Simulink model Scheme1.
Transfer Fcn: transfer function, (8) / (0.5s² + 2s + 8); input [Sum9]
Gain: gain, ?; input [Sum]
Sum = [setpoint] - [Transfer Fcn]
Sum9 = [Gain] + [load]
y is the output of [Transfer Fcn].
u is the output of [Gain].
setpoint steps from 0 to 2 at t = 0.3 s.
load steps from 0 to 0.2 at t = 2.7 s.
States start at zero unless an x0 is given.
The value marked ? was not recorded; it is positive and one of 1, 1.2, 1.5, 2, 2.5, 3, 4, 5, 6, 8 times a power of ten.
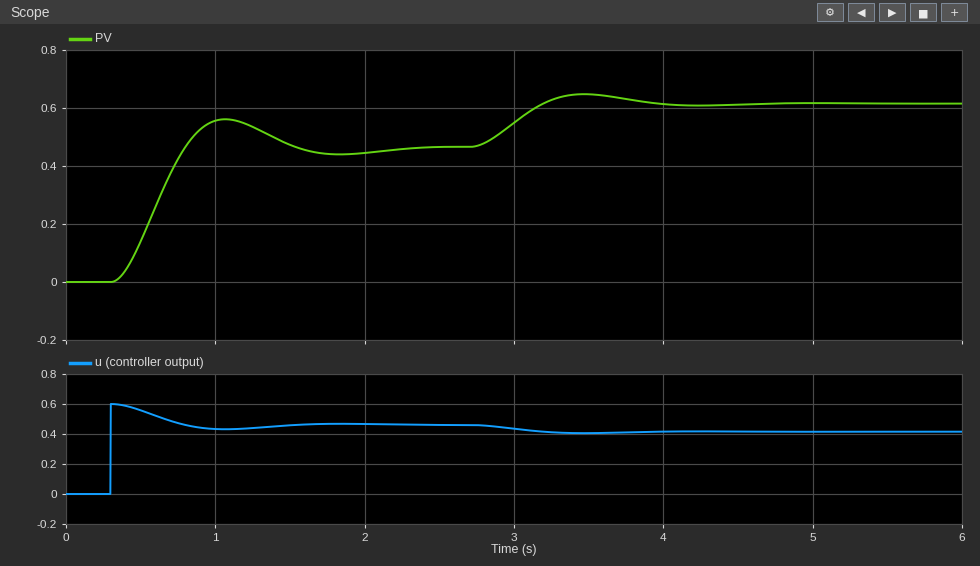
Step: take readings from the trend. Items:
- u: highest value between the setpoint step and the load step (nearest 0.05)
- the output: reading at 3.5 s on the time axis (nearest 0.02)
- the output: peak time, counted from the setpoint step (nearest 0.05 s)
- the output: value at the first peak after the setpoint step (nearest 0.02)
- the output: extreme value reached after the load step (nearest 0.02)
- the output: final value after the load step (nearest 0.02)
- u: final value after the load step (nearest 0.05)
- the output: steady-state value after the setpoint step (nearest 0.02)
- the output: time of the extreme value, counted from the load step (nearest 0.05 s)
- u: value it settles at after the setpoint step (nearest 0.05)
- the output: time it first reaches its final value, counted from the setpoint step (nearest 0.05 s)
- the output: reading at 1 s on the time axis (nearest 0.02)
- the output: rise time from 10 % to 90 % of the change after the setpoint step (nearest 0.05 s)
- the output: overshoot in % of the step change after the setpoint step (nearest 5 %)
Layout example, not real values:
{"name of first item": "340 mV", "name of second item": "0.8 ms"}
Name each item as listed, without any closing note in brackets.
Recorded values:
{"u: highest value between the setpoint step and the load step": "0.60", "the output: reading at 3.5 s on the time axis": "0.64", "the output: peak time, counted from the setpoint step": "0.75 s", "the output: value at the first peak after the setpoint step": "0.56", "the output: extreme value reached after the load step": "0.64", "the output: final value after the load step": "0.62", "u: final value after the load step": "0.40", "the output: steady-state value after the setpoint step": "0.46", "the output: time of the extreme value, counted from the load step": "0.75 s", "u: value it settles at after the setpoint step": "0.45", "the output: time it first reaches its final value, counted from the setpoint step": "0.50 s", "the output: reading at 1 s on the time axis": "0.56", "the output: rise time from 10 % to 90 % of the change after the setpoint step": "0.35 s", "the output: overshoot in % of the step change after the setpoint step": "20 %"}
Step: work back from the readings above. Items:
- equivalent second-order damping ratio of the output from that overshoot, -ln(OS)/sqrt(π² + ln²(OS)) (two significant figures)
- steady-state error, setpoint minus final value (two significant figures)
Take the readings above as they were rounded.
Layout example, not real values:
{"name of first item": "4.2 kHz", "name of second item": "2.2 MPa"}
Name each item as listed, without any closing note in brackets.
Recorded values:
{"equivalent second-order damping ratio of the output from that overshoot, -ln(OS)/sqrt(π² + ln²(OS))": "0.46", "steady-state error, setpoint minus final value": "1.5"}
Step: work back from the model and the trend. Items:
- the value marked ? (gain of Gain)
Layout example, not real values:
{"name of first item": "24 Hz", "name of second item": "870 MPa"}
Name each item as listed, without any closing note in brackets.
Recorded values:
{"the value marked ?": "0.3"}
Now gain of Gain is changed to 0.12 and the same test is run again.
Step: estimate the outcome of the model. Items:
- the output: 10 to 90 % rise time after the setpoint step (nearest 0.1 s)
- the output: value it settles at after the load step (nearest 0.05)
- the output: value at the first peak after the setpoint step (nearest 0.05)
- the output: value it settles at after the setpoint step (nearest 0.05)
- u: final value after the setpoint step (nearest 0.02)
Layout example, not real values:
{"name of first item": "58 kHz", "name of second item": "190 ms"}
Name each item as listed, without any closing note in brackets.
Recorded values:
{"the output: 10 to 90 % rise time after the setpoint step": "0.4 s", "the output: value it settles at after the load step": "0.40", "the output: value at the first peak after the setpoint step": "0.25", "the output: value it settles at after the setpoint step": "0.20", "u: final value after the setpoint step": "0.22"}
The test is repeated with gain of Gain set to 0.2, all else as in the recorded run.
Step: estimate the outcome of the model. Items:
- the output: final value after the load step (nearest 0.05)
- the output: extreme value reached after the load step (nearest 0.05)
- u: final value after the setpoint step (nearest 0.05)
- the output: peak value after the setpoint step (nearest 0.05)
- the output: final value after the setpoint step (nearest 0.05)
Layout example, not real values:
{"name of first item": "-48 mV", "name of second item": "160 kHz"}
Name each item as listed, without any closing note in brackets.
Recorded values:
{"the output: final value after the load step": "0.50", "the output: extreme value reached after the load step": "0.55", "u: final value after the setpoint step": "0.35", "the output: peak value after the setpoint step": "0.40", "the output: final value after the setpoint step": "0.35"}
